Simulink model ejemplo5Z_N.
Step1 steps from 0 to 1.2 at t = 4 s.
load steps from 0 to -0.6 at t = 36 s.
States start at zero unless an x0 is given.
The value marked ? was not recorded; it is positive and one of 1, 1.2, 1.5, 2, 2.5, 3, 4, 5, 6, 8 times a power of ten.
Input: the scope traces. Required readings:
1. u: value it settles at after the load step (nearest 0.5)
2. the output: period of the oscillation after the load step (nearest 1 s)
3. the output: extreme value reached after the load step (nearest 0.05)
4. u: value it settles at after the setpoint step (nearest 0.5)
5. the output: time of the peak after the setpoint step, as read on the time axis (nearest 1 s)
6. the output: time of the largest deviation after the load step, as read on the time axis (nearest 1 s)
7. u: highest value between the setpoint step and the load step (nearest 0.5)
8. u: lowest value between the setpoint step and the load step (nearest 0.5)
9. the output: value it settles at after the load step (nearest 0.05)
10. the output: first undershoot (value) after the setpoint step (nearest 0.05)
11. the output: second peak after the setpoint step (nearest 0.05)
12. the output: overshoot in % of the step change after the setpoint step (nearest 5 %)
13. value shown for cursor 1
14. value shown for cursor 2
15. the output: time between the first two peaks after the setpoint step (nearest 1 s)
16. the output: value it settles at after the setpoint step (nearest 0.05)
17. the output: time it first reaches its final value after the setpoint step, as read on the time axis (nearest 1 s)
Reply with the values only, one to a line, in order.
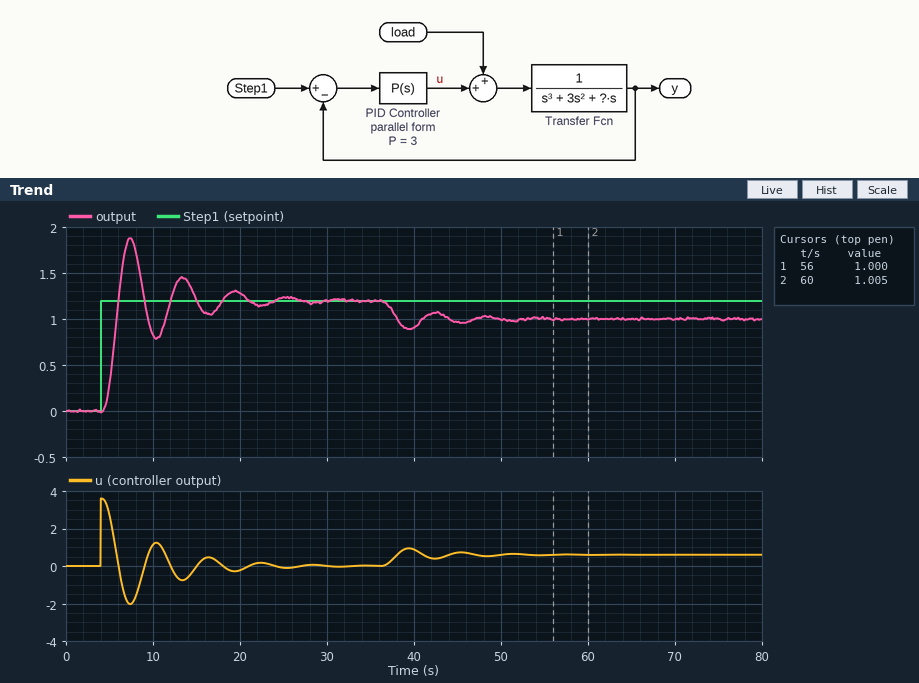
0.5
6 s
0.90
0.0
7 s
39 s
3.5
-2.0
1.00
0.80
1.45
55 %
1.000
1.005
6 s
1.20
6 s
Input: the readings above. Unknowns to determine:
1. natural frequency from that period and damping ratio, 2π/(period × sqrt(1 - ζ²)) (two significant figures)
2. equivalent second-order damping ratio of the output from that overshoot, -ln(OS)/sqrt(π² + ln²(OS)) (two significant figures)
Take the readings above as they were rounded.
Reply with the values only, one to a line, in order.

1.1 rad/s
0.19
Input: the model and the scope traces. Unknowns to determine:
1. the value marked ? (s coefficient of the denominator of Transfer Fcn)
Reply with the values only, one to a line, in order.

2
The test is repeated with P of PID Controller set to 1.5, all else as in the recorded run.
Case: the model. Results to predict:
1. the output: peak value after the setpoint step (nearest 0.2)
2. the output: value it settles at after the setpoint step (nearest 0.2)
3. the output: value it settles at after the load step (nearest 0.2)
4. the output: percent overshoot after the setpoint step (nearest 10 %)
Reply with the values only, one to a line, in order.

1.6
1.2
0.8
30 %
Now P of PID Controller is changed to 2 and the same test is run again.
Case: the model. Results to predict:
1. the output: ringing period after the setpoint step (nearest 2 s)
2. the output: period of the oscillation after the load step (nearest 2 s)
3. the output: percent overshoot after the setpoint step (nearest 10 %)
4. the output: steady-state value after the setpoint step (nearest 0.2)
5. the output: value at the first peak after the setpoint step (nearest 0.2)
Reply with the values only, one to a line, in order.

8 s
8 s
40 %
1.2
1.6
